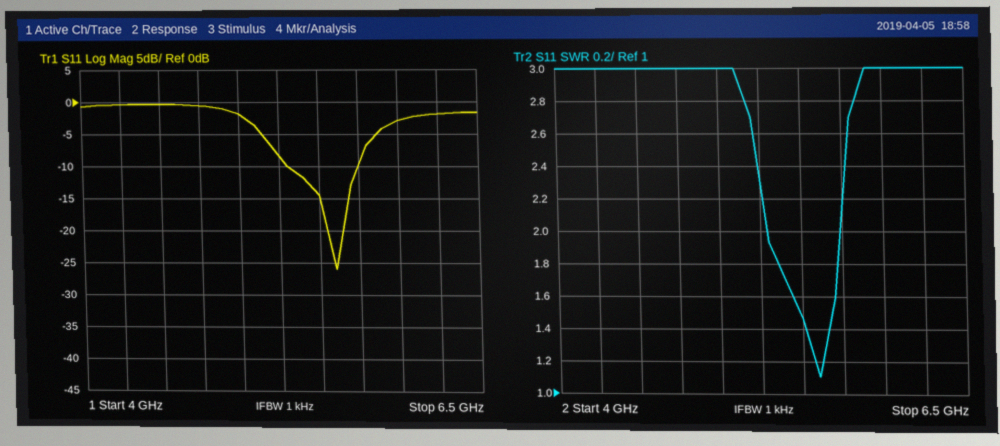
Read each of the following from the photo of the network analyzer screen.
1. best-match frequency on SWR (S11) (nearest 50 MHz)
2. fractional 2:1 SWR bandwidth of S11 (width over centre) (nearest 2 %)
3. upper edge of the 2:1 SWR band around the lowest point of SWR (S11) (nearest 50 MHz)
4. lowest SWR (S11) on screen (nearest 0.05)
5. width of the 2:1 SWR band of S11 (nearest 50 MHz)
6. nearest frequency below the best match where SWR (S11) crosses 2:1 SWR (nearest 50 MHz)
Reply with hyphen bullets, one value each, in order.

- 5.60 GHz
- 8 %
- 5.75 GHz
- 1.10
- 450 MHz
- 5.30 GHz
